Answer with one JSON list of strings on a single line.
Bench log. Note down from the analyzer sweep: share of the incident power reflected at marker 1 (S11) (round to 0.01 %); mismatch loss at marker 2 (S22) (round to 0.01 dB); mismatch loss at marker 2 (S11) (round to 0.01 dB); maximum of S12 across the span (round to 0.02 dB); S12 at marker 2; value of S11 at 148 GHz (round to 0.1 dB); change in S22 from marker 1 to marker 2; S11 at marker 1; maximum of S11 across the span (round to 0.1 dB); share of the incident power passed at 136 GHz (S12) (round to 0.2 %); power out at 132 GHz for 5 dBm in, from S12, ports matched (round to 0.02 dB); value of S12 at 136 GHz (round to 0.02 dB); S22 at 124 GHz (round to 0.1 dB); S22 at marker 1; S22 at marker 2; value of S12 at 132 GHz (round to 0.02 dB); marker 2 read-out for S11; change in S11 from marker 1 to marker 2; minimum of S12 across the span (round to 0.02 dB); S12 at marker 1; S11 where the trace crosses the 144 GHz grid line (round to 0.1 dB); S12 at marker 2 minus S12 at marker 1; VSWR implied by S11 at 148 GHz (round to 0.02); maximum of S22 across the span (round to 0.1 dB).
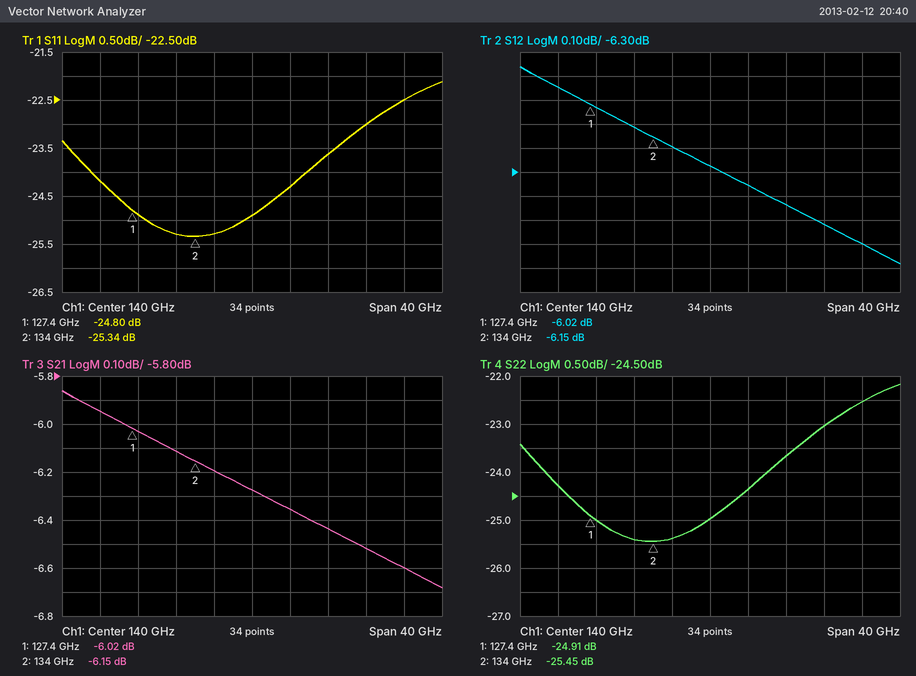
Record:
["0.33 %", "0.01 dB", "0.01 dB", "-5.86 dB", "-6.15 dB", "-23.6 dB", "-0.54 dB", "-24.80 dB", "-22.1 dB", "24.0 %", "-1.12 dBm", "-6.20 dB", "-24.3 dB", "-24.91 dB", "-25.45 dB", "-6.12 dB", "-25.34 dB", "-0.54 dB", "-6.68 dB", "-6.02 dB", "-24.3 dB", "-0.13 dB", "1.14", "-22.2 dB"]
